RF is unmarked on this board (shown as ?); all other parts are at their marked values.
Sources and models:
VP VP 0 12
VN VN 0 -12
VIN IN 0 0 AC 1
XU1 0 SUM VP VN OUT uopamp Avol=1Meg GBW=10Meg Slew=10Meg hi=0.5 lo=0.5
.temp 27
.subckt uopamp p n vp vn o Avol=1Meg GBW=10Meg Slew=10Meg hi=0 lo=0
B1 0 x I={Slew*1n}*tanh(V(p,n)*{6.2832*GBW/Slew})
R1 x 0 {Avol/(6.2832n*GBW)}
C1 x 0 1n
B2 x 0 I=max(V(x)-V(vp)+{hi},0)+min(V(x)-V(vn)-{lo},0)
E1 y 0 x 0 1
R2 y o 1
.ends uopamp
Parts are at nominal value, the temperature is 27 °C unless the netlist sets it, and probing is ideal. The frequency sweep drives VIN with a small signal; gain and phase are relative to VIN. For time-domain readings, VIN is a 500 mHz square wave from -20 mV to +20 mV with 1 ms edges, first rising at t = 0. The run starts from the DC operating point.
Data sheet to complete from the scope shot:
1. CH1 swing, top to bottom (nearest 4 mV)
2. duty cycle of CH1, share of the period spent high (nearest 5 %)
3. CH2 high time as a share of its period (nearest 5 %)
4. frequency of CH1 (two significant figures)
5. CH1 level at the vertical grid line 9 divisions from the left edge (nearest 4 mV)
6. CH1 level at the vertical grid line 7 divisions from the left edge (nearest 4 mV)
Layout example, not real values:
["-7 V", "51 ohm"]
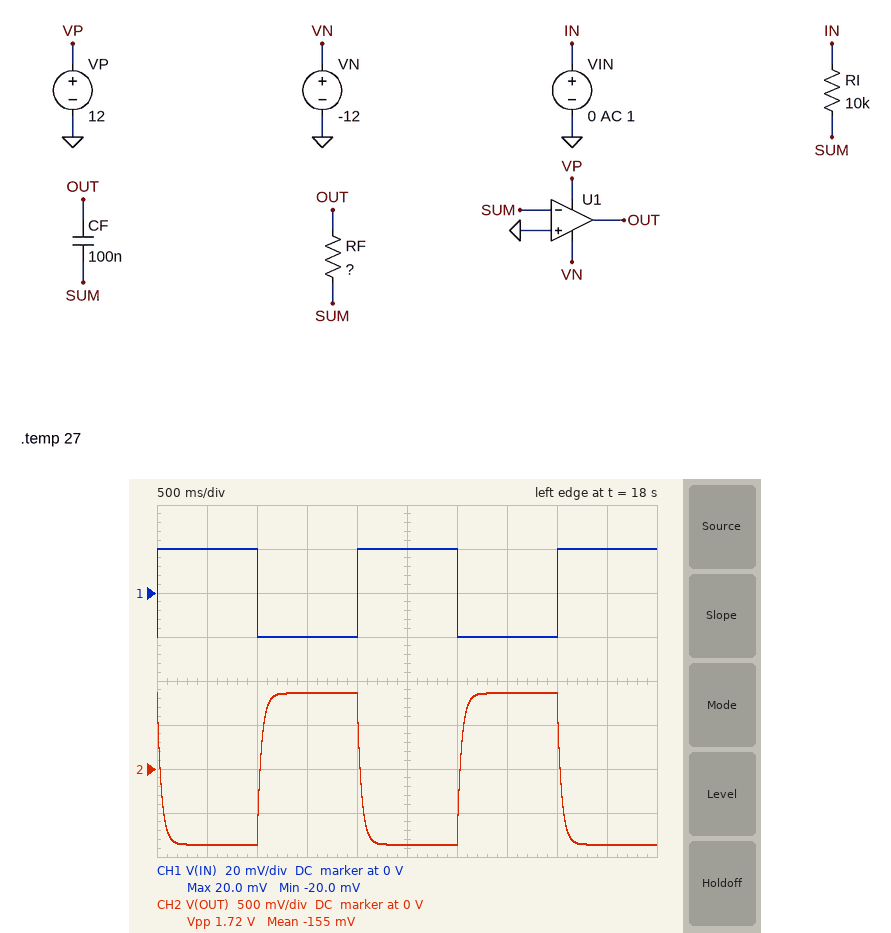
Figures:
["40 mV", "50 %", "50 %", "500 mHz", "20 mV", "-20 mV"]
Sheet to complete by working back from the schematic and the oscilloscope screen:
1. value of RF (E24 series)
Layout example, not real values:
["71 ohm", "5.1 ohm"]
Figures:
["430 kΩ"]
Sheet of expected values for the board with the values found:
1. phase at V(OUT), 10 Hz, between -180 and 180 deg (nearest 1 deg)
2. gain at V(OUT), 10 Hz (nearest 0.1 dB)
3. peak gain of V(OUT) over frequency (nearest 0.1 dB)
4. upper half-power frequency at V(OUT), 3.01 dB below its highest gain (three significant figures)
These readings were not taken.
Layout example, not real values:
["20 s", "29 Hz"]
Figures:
["110 deg", "23.5 dB", "32.7 dB", "3.70 Hz"]
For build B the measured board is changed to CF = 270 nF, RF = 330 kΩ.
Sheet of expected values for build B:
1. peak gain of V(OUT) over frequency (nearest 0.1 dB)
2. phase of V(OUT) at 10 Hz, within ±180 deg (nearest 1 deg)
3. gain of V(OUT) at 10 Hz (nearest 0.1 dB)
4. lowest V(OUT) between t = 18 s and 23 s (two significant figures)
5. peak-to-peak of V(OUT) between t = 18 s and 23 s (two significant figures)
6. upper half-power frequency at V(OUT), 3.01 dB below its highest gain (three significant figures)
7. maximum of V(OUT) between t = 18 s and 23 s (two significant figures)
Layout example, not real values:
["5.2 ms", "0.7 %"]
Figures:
["30.4 dB", "100 deg", "15.3 dB", "-660 mV", "1.3 V", "1.79 Hz", "660 mV"]
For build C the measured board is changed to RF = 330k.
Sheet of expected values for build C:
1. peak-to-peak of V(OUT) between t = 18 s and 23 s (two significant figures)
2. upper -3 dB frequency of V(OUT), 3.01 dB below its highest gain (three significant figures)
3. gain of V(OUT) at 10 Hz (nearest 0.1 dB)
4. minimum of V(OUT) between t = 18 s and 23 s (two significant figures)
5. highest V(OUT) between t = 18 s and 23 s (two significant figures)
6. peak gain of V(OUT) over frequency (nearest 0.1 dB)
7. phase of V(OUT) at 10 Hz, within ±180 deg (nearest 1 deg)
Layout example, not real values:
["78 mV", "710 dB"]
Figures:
["1.3 V", "4.82 Hz", "23.1 dB", "-660 mV", "660 mV", "30.4 dB", "116 deg"]
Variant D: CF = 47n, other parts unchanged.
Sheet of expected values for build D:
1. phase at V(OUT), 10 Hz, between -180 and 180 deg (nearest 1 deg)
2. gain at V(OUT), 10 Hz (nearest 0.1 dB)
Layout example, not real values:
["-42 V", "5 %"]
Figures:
["128 deg", "28.5 dB"]
